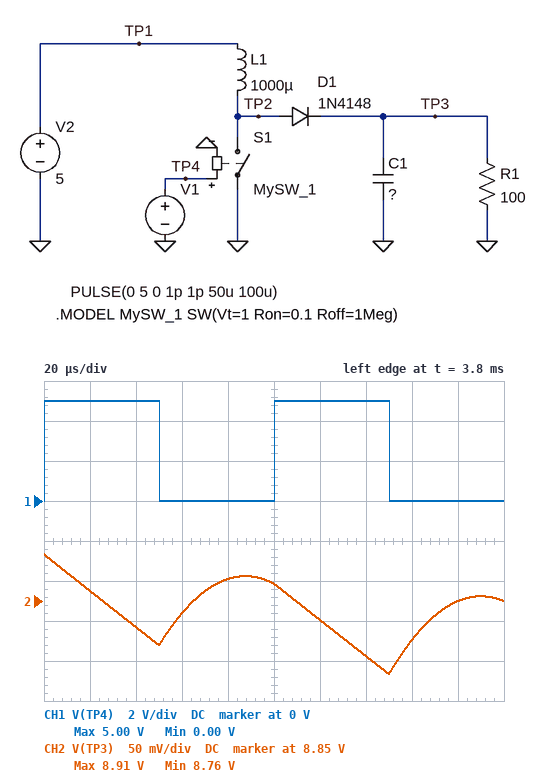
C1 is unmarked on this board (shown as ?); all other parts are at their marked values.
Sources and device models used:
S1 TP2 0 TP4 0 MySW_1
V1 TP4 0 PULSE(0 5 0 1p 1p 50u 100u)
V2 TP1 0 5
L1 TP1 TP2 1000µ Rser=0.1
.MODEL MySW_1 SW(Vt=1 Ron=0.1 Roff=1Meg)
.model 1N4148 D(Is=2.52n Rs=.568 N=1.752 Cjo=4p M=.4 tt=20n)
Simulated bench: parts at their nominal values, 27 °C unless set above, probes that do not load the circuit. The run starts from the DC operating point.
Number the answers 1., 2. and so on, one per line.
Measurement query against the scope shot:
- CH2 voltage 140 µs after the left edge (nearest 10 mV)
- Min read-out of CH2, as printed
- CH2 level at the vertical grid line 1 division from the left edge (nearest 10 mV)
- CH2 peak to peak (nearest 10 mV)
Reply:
1. 8.78 V
2. 8.76 V
3. 8.86 V
4. 150 mV
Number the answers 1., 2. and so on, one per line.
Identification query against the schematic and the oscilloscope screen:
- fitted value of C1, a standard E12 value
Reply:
1. 39 µF
